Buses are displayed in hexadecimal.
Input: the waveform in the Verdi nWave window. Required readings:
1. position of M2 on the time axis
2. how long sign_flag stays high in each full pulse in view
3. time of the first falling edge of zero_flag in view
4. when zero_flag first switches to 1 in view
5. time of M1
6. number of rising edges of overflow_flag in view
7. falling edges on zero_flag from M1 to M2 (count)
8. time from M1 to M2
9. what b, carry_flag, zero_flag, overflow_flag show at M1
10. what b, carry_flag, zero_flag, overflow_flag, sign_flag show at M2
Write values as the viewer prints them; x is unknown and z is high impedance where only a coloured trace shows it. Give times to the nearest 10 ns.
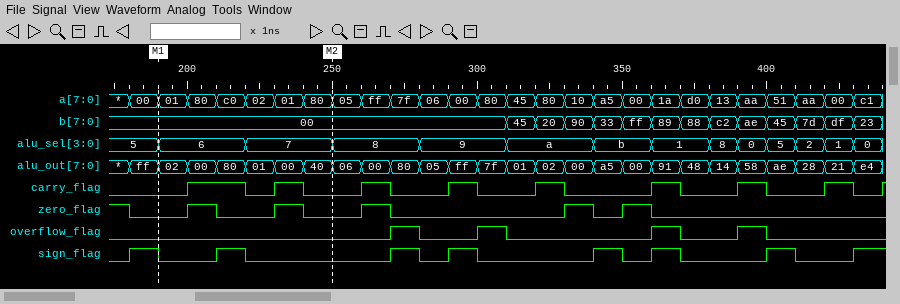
250 ns
10 ns, 10 ns, 10 ns, 10 ns, 10 ns, 10 ns, 10 ns
180 ns
200 ns
190 ns
4
2
60 ns
b=00, carry_flag=0, zero_flag=0, overflow_flag=0
b=00, carry_flag=0, zero_flag=0, overflow_flag=0, sign_flag=0
